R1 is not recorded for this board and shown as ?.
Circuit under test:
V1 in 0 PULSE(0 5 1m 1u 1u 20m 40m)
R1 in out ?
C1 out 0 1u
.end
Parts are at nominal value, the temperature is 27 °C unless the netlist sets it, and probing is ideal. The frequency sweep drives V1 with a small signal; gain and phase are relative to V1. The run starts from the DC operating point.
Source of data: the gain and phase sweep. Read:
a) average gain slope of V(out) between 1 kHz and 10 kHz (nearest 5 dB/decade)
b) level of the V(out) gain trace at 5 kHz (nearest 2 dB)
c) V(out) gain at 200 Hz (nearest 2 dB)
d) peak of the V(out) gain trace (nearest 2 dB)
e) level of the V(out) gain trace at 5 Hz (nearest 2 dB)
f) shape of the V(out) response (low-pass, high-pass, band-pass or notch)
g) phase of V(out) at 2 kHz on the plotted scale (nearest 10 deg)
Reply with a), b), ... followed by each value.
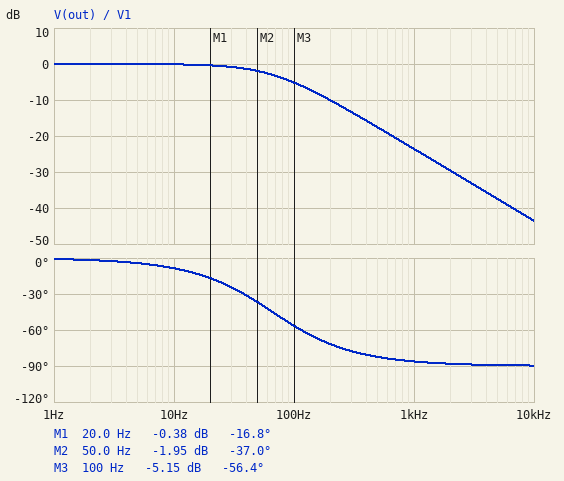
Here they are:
a) -20 dB/decade
b) -38 dB
c) -10 dB
d) 0 dB
e) 0 dB
f) low-pass
g) -90 deg
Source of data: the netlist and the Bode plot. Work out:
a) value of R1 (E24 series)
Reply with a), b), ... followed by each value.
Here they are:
a) 2.4 kΩ
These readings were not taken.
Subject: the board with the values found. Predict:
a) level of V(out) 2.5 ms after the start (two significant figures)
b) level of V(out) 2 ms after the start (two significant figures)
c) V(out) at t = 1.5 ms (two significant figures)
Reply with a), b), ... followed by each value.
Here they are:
a) 2.3 V
b) 1.7 V
c) 940 mV
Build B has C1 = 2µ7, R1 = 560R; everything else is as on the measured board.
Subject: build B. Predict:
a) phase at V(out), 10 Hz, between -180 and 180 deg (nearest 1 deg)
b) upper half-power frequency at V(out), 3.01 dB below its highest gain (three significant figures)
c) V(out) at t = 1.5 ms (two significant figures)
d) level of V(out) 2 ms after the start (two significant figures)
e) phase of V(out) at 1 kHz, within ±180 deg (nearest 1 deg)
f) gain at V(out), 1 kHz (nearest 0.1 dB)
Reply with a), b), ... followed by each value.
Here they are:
a) -5 deg
b) 105 Hz
c) 1.4 V
d) 2.4 V
e) -84 deg
f) -19.6 dB
